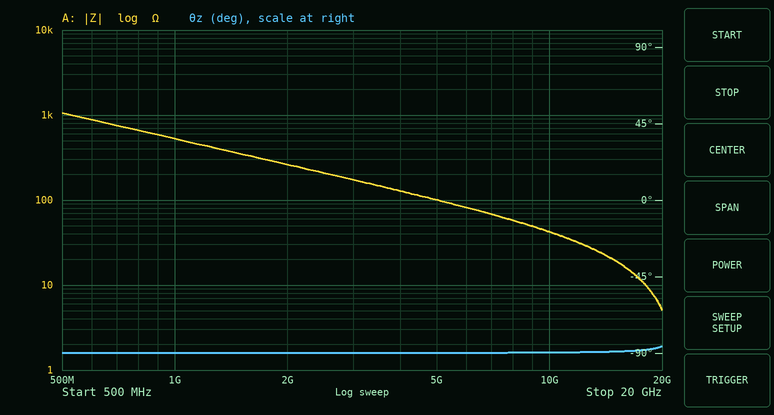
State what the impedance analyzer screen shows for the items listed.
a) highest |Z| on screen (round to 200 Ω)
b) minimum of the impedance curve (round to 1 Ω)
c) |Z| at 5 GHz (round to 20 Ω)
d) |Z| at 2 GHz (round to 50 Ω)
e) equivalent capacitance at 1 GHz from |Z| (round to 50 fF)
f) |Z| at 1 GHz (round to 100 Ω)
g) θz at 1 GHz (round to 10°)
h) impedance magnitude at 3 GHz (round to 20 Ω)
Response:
1.0 kΩ
5 Ω
100 Ω
250 Ω
300 fF
500 Ω
-90°
180 Ω
